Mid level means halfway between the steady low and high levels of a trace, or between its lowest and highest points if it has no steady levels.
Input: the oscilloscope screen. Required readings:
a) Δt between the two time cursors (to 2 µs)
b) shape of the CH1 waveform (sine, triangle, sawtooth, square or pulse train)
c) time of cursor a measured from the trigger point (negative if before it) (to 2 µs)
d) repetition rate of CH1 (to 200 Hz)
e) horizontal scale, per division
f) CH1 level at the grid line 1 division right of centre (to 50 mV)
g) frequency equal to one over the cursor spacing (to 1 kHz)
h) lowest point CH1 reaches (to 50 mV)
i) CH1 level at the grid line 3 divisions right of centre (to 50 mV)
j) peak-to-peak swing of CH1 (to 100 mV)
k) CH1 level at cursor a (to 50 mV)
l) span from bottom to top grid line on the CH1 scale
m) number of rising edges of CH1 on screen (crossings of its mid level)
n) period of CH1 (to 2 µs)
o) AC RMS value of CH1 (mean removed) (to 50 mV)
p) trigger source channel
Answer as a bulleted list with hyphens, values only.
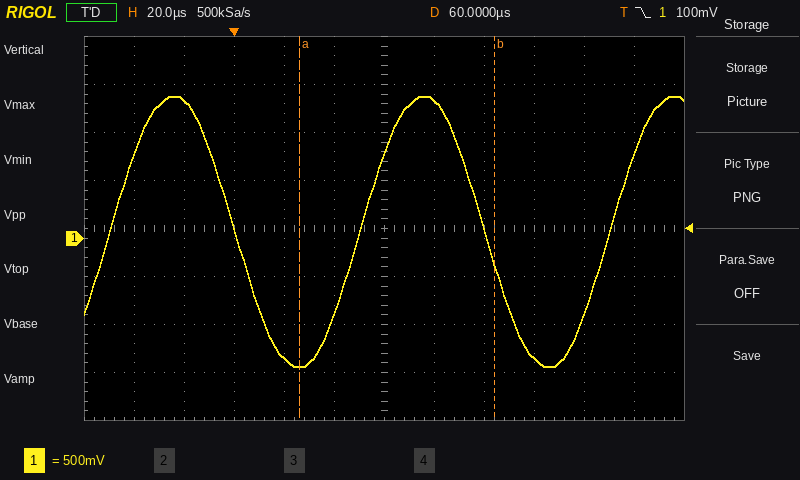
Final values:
- 78 µs
- sine
- +26 µs
- 10.0 kHz
- 20 µs
- 1.45 V
- 13 kHz
- -1.35 V
- -1.25 V
- 2.80 V
- -1.35 V
- 4 V
- 3
- 100 µs
- 1.00 V
- CH1
